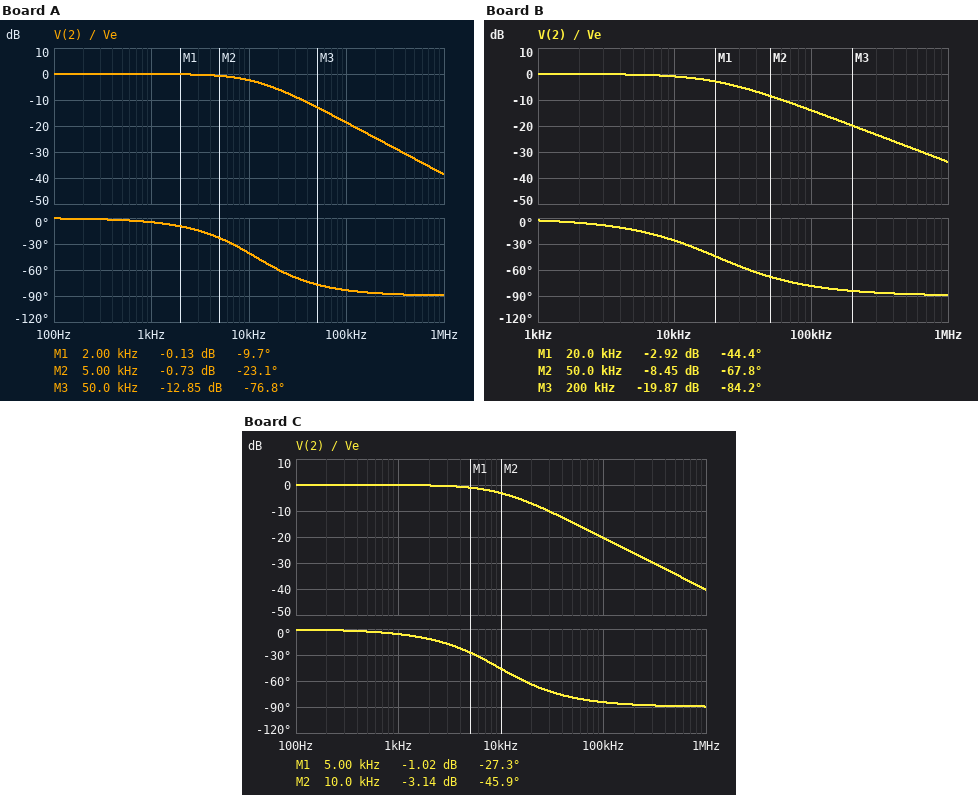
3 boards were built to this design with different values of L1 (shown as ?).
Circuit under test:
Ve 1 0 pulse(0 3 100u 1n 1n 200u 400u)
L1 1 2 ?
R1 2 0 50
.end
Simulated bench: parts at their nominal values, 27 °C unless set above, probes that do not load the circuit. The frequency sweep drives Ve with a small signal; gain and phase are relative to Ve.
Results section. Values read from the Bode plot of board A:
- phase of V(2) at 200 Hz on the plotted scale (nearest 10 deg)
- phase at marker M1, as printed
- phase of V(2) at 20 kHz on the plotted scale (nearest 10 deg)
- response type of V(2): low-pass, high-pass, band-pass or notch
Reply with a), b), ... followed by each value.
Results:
a) 0 deg
b) -9.7 deg
c) -60 deg
d) low-pass
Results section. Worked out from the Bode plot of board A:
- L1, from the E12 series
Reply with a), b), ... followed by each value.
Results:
a) 680 µH
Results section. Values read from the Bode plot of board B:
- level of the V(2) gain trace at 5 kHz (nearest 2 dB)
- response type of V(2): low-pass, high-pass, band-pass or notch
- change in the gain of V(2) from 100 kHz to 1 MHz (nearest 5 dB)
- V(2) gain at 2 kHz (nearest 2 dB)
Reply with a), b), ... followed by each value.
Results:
a) 0 dB
b) low-pass
c) -20 dB
d) 0 dB
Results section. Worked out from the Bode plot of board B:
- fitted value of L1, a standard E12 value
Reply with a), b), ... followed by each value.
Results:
a) 390 µH
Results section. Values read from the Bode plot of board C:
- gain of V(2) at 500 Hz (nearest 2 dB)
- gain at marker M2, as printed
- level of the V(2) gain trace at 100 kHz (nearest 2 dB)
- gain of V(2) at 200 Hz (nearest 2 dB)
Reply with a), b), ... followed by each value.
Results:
a) 0 dB
b) -3.14 dB
c) -20 dB
d) 0 dB
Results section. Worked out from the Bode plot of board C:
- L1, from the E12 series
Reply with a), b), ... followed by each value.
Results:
a) 820 µH
